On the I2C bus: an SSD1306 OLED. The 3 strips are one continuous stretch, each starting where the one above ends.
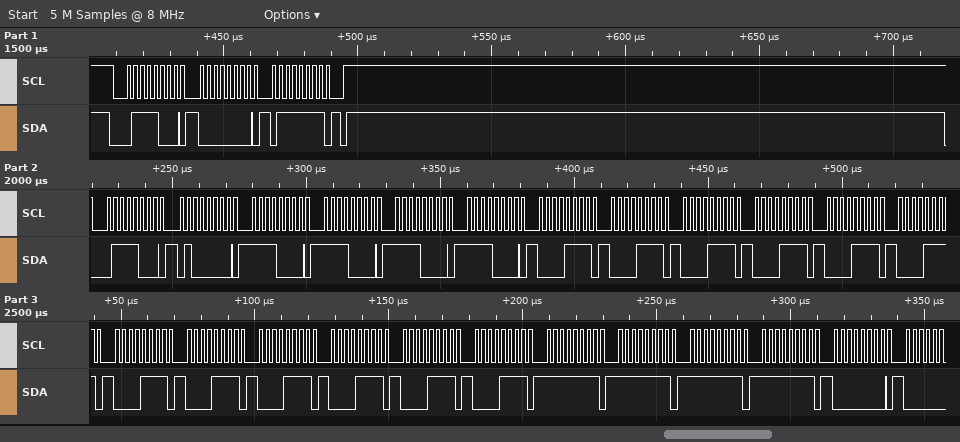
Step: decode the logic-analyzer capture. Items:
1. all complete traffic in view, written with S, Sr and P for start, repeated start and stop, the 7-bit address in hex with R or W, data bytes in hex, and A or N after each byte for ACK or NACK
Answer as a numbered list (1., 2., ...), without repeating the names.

1. S 3CW A 00 A 7F A P S 3CW A 40 A F0 A F0 A F0 A F0 A 0F A 0F A 0F A 0F A 0F A 0F A 0F A 0F A 0F A 0F A 0F A 0F A FF A FF A FF A FF A 00 A
